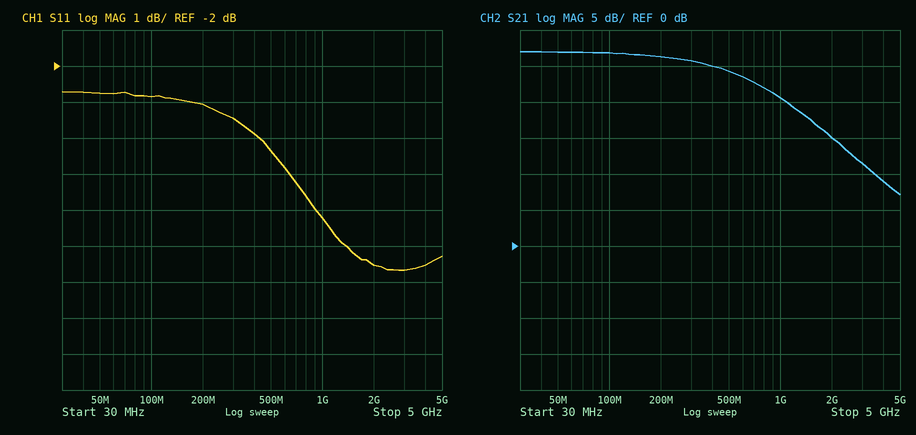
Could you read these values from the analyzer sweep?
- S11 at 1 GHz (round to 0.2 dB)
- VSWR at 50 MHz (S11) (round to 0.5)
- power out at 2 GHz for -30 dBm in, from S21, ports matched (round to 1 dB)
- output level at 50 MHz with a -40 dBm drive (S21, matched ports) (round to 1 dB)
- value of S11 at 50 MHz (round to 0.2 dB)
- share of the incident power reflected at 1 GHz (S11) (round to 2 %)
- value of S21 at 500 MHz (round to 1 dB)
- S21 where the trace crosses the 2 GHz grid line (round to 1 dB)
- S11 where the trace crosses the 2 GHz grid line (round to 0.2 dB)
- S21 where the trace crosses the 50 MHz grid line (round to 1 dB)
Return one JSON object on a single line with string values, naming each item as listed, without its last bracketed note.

{"S11 at 1 GHz": "-6.2 dB", "VSWR at 50 MHz (S11)": "6.5", "power out at 2 GHz for -30 dBm in, from S21, ports matched": "-15 dBm", "output level at 50 MHz with a -40 dBm drive (S21, matched ports)": "-13 dBm", "value of S11 at 50 MHz": "-2.8 dB", "share of the incident power reflected at 1 GHz (S11)": "24 %", "value of S21 at 500 MHz": "24 dB", "S21 where the trace crosses the 2 GHz grid line": "15 dB", "S11 where the trace crosses the 2 GHz grid line": "-7.6 dB", "S21 where the trace crosses the 50 MHz grid line": "27 dB"}
